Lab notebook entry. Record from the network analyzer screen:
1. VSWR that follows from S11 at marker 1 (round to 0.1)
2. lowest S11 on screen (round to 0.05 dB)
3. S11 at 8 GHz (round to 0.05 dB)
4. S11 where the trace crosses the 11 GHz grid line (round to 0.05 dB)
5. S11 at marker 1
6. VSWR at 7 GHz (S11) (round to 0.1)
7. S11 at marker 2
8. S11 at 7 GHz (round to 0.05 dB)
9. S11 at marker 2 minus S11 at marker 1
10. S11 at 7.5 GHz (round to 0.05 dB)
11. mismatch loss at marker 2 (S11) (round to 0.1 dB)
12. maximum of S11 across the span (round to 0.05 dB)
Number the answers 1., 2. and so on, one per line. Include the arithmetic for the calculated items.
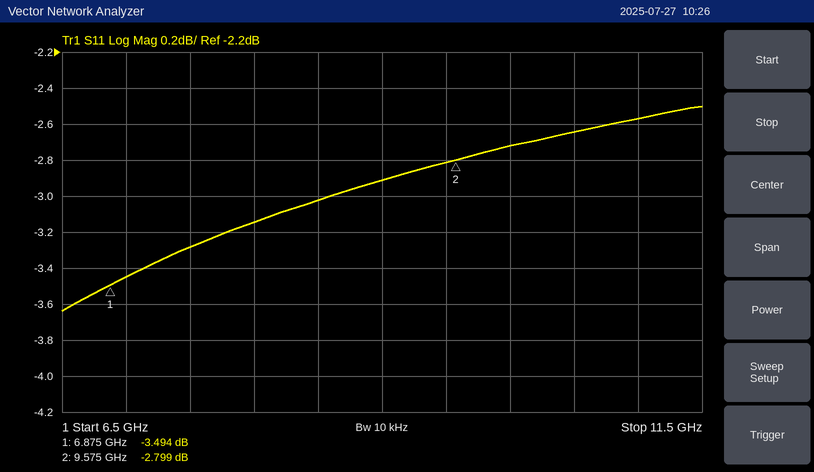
1. (1 + 0.6688)/(1 − 0.6688) ≈ 5.0
2. -3.65 dB
3. -3.15 dB
4. -2.55 dB
5. -3.494 dB
6. |Γ| = 10^(-3.45/20) = 0.6722; VSWR = (1 + 0.6722)/(1 − 0.6722) ≈ 5.1
7. -2.799 dB
8. -3.45 dB
9. -2.799 − (-3.494) = 0.695 dB
10. -3.30 dB
11. −10 log10(1 − 10^(-2.799/10)) ≈ 3.2 dB
12. -2.50 dB
